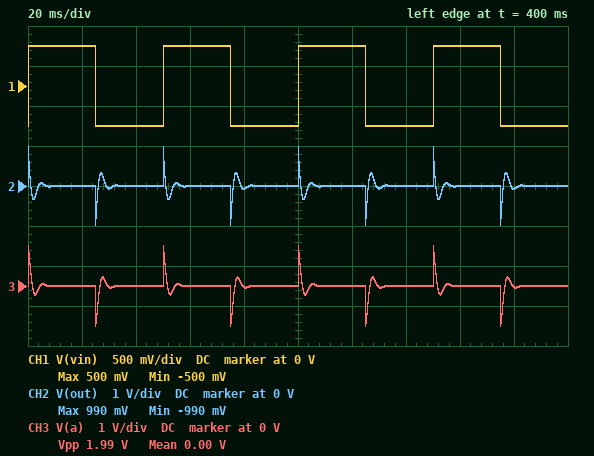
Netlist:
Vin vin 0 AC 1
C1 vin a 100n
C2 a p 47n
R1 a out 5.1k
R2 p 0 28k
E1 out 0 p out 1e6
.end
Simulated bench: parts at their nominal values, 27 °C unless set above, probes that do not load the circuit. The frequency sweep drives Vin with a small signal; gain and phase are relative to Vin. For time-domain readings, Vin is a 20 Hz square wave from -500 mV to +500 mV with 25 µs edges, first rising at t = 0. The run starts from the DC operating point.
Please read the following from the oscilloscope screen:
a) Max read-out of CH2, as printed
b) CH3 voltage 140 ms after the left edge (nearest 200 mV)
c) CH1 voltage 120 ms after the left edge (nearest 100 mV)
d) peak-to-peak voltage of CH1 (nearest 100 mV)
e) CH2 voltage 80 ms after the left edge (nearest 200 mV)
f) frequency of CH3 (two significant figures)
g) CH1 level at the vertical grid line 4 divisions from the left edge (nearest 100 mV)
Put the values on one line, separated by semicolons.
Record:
990 mV; 0 V; 500 mV; 1.0 V; 0 V; 20 Hz; -500 mV
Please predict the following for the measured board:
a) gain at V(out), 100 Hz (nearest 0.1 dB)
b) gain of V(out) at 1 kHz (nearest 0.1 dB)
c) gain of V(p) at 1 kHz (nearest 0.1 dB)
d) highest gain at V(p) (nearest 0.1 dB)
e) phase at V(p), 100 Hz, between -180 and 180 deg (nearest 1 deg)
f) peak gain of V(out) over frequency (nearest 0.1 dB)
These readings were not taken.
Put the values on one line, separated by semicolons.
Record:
-10.4 dB; 0.2 dB; 0.2 dB; 1.8 dB; 147 deg; 1.8 dB
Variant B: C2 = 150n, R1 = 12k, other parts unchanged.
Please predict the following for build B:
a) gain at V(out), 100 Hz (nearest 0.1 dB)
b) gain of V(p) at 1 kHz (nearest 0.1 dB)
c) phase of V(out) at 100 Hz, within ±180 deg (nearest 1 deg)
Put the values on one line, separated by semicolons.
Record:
-0.6 dB; 0 dB; 62 deg
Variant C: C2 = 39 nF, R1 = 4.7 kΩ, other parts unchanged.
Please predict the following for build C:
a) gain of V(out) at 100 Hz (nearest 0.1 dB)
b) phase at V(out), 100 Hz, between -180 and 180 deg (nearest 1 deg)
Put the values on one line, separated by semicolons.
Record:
-12.9 dB; 153 deg
